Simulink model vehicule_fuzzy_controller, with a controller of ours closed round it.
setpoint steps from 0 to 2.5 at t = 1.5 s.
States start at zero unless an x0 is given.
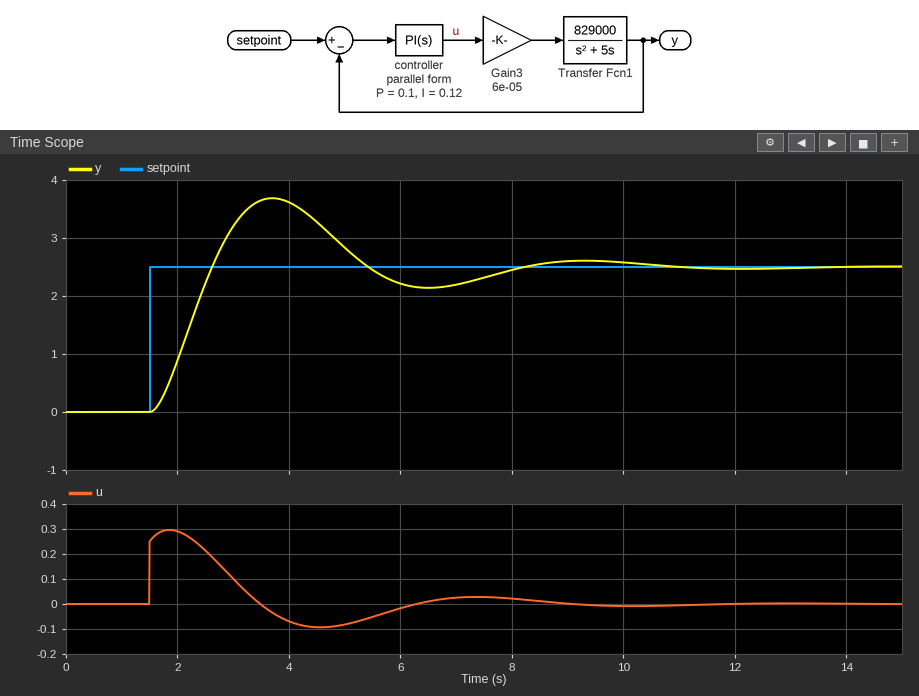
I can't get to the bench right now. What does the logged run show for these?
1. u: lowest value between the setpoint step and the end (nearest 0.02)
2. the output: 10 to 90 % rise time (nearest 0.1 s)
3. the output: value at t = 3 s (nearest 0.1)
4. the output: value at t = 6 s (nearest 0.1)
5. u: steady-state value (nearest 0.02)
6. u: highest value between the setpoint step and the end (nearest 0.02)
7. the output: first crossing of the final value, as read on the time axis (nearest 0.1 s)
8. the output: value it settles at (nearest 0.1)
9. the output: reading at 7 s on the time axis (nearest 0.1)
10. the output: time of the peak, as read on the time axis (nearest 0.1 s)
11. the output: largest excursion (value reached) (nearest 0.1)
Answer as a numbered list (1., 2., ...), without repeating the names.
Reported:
1. -0.10
2. 0.8 s
3. 3.2
4. 2.2
5. 0.00
6. 0.30
7. 2.6 s
8. 2.5
9. 2.2
10. 3.7 s
11. 3.7
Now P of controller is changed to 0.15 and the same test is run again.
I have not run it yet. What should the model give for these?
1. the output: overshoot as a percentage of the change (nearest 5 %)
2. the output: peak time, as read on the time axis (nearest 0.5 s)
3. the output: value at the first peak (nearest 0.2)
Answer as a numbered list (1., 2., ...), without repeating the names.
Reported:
1. 35 %
2. 3.5 s
3. 3.4
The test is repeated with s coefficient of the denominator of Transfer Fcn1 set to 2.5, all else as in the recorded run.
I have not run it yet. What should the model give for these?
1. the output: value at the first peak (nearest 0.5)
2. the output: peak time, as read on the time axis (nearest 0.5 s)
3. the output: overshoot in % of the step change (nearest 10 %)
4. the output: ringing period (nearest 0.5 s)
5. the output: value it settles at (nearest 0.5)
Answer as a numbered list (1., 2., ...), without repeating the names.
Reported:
1. 4.0
2. 3.0 s
3. 70 %
4. 3.5 s
5. 2.5
